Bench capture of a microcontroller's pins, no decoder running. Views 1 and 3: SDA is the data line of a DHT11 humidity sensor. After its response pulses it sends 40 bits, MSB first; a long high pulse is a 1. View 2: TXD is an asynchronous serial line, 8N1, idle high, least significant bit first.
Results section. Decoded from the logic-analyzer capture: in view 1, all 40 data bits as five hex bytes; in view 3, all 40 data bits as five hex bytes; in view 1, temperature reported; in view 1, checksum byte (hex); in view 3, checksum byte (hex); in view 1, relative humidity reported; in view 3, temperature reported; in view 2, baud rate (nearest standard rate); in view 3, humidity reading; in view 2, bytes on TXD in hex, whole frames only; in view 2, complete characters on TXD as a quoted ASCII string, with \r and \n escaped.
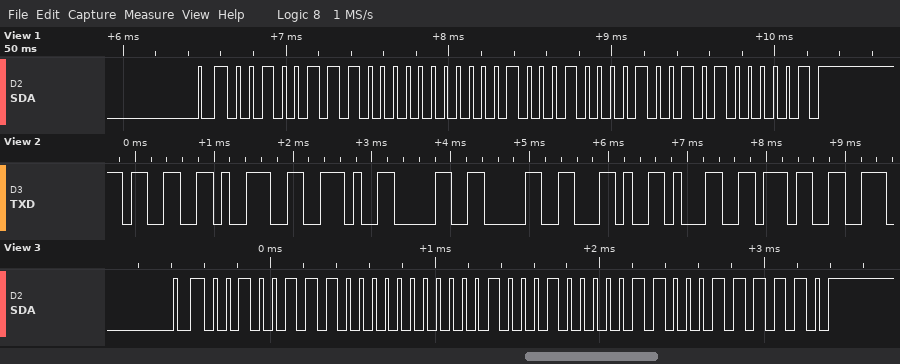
27 00 11 09 41
27 00 11 06 3E
17.9 °C
0x41
0x3E
39 %
17.6 °C
9600 baud
39 %
0x33 0x39 0x2E 0x30 0x30 0x2C 0x31 0x37
"39.00,17"
